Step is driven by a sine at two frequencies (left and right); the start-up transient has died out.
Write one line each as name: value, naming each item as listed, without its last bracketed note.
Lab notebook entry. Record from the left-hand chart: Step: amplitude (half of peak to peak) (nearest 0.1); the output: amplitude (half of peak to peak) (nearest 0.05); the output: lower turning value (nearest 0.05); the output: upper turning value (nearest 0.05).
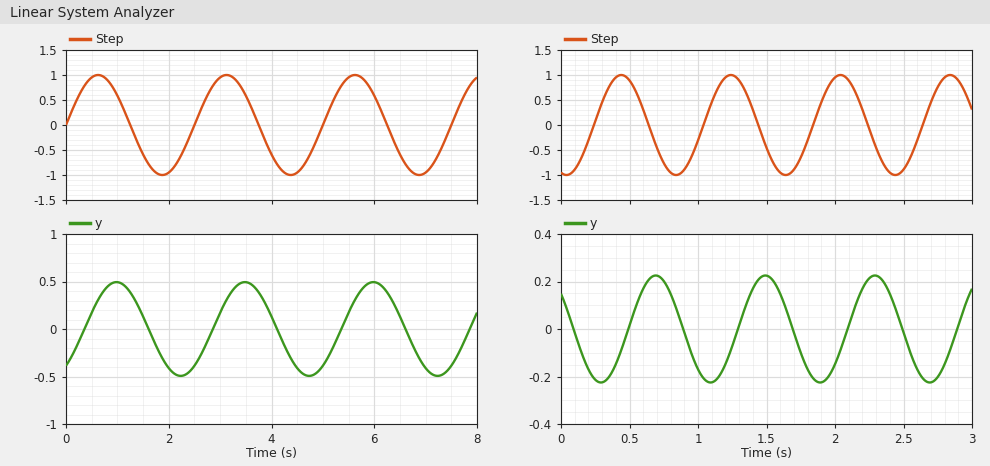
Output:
Step: amplitude (half of peak to peak): 1.0
the output: amplitude (half of peak to peak): 0.50
the output: lower turning value: -0.50
the output: upper turning value: 0.50
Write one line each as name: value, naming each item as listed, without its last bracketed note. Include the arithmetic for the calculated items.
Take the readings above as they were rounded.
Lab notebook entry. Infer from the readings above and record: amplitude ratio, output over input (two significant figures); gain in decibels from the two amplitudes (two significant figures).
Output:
amplitude ratio, output over input: 0.5 / 1 = 0.50
gain in decibels from the two amplitudes: 20 log10(0.5 / 1) = -6.0 dB
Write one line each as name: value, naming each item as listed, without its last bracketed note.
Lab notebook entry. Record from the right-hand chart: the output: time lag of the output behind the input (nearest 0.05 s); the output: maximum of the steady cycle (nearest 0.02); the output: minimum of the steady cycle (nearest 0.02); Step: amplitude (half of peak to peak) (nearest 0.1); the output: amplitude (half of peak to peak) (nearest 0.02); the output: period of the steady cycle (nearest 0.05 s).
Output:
the output: time lag of the output behind the input: 0.25 s
the output: maximum of the steady cycle: 0.22
the output: minimum of the steady cycle: -0.22
Step: amplitude (half of peak to peak): 1.0
the output: amplitude (half of peak to peak): 0.22
the output: period of the steady cycle: 0.80 s
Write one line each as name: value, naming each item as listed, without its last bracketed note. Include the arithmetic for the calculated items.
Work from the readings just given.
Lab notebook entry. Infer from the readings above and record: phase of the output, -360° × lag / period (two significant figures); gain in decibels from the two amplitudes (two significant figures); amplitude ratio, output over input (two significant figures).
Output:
phase of the output, -360° × lag / period: -360 × 0.25 / 0.8 = -110°
gain in decibels from the two amplitudes: 20 log10(0.22 / 1) = -13 dB
amplitude ratio, output over input: 0.22 / 1 = 0.22
